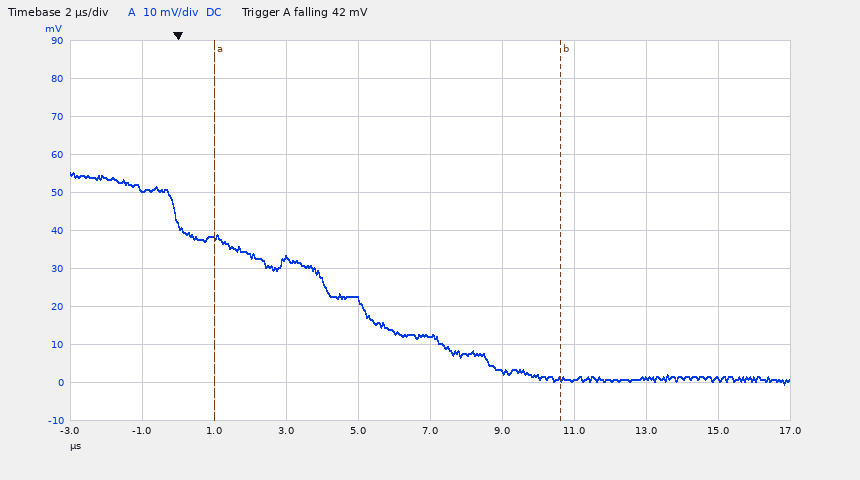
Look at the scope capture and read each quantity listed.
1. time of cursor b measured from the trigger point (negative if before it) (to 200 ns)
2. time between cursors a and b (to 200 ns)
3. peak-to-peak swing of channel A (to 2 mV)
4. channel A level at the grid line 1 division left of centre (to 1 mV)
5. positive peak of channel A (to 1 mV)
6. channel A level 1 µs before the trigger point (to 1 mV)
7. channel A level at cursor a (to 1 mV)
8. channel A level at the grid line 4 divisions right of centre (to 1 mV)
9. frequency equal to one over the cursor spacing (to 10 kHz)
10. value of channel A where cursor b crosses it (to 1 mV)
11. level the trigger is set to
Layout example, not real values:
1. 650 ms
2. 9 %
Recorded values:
1. +10.6 µs
2. 9.6 µs
3. 56 mV
4. 22 mV
5. 55 mV
6. 51 mV
7. 38 mV
8. 1 mV
9. 100 kHz
10. 1 mV
11. 42 mV
